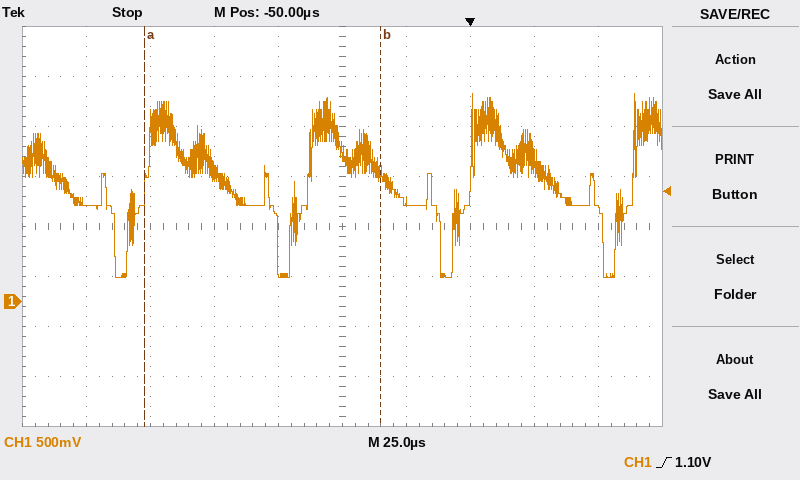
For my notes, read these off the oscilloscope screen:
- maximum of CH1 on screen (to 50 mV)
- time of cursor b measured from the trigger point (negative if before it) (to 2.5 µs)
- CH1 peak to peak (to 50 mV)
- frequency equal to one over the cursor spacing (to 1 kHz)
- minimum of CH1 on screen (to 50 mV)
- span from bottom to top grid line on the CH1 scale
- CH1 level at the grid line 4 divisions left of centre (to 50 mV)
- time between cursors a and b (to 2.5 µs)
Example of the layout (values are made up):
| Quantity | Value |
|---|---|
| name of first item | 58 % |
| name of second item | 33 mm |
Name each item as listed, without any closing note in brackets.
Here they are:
| Quantity | Value |
|---|---|
| maximum of CH1 on screen | 2.10 V |
| time of cursor b measured from the trigger point (negative if before it) | -35.0 µs |
| CH1 peak to peak | 1.85 V |
| frequency equal to one over the cursor spacing | 11 kHz |
| minimum of CH1 on screen | 250 mV |
| span from bottom to top grid line on the CH1 scale | 4 V |
| CH1 level at the grid line 4 divisions left of centre | 950 mV |
| time between cursors a and b | 92.5 µs |
